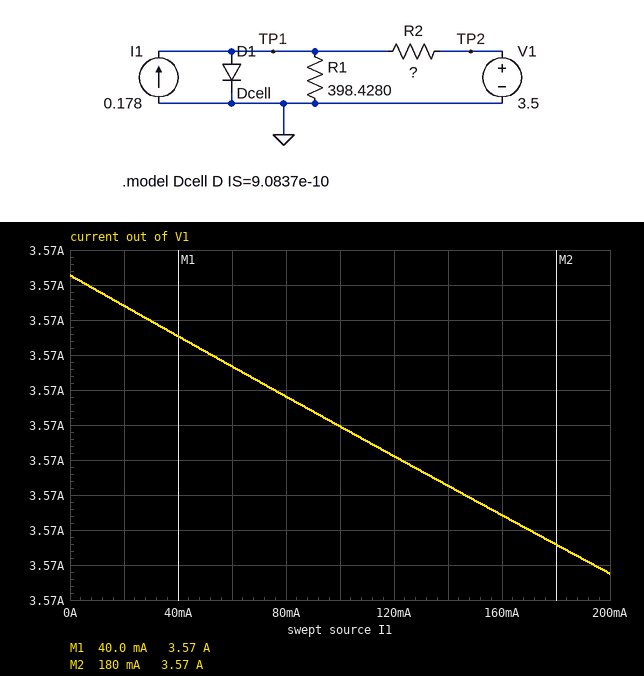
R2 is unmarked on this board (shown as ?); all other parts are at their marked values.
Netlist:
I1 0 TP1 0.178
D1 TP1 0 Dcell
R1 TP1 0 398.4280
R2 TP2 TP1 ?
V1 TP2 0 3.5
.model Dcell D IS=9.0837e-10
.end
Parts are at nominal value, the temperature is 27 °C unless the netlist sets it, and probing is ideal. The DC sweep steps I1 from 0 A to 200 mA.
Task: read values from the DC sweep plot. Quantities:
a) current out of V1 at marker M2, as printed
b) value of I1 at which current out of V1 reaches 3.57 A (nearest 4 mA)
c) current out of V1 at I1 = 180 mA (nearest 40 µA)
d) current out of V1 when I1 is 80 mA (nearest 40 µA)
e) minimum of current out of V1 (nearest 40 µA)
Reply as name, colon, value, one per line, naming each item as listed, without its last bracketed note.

current out of V1 at marker M2, as printed: 3.57 A
value of I1 at which current out of V1 reaches 3.57 A: 76 mA
current out of V1 at I1 = 180 mA: 3.56992 A
current out of V1 when I1 is 80 mA: 3.57076 A
minimum of current out of V1: 3.56976 A
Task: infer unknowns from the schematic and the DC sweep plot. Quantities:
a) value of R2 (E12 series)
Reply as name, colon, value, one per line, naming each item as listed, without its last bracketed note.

value of R2: 0.82 Ω
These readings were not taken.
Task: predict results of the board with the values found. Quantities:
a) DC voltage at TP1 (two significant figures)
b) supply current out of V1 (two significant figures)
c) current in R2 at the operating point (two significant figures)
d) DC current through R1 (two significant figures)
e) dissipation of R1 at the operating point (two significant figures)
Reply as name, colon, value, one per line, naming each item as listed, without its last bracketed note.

DC voltage at TP1: 570 mV
supply current out of V1: 3.6 A
current in R2 at the operating point: 3.6 A
DC current through R1: 1.4 mA
dissipation of R1 at the operating point: 820 µW
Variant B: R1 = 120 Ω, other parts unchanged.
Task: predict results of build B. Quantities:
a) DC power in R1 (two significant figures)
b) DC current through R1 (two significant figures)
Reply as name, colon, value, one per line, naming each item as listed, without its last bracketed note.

DC power in R1: 2.7 mW
DC current through R1: 4.8 mA
